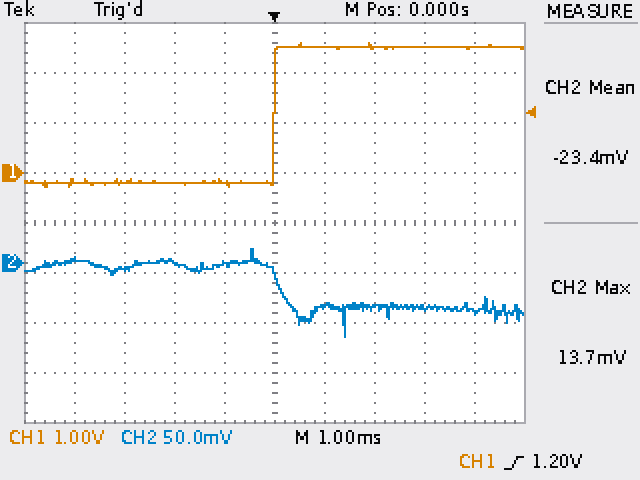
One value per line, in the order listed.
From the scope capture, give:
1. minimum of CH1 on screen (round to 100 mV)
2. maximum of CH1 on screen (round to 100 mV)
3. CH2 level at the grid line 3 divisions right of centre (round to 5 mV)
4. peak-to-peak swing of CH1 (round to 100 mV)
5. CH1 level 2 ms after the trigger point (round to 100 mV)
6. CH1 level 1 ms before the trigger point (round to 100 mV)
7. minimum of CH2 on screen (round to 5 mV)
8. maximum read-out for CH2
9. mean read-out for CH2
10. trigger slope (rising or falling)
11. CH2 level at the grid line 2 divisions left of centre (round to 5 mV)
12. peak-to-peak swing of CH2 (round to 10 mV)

-300 mV
2.6 V
-45 mV
2.9 V
2.5 V
-200 mV
-75 mV
13.7 mV
-23.4 mV
rising
0 mV
90 mV
